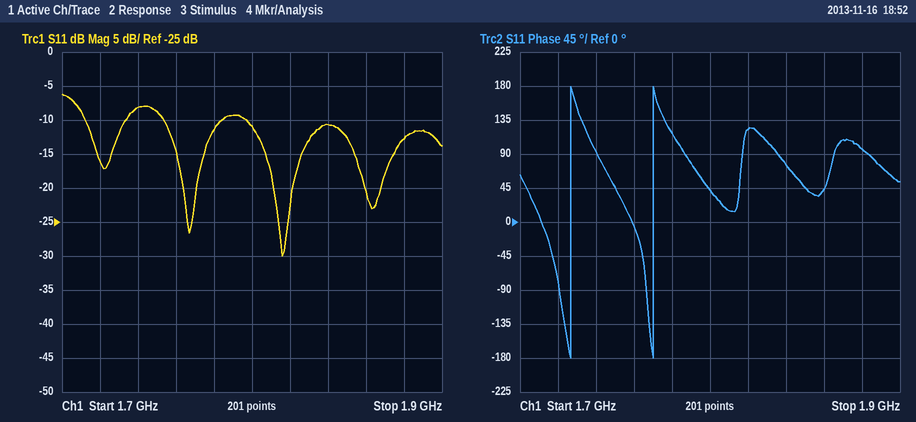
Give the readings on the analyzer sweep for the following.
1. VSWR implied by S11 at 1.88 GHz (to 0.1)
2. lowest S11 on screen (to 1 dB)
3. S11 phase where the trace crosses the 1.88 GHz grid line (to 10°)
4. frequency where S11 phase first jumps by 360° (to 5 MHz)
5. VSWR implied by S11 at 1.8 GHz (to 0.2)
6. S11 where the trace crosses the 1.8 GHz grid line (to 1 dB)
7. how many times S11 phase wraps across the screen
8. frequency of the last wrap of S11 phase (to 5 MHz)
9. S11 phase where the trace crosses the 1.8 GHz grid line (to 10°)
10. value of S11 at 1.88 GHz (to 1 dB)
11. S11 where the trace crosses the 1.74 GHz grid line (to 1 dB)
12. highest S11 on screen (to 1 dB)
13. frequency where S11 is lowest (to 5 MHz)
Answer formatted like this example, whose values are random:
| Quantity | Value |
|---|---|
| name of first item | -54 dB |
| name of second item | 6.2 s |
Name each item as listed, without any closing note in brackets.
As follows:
| Quantity | Value |
|---|---|
| VSWR implied by S11 at 1.88 GHz | 1.6 |
| lowest S11 on screen | -30 dB |
| S11 phase where the trace crosses the 1.88 GHz grid line | 100° |
| frequency where S11 phase first jumps by 360° | 1.725 GHz |
| VSWR implied by S11 at 1.8 GHz | 1.8 |
| S11 where the trace crosses the 1.8 GHz grid line | -11 dB |
| how many times S11 phase wraps across the screen | 2 |
| frequency of the last wrap of S11 phase | 1.770 GHz |
| S11 phase where the trace crosses the 1.8 GHz grid line | 40° |
| value of S11 at 1.88 GHz | -13 dB |
| S11 where the trace crosses the 1.74 GHz grid line | -8 dB |
| highest S11 on screen | -6 dB |
| frequency where S11 is lowest | 1.815 GHz |
